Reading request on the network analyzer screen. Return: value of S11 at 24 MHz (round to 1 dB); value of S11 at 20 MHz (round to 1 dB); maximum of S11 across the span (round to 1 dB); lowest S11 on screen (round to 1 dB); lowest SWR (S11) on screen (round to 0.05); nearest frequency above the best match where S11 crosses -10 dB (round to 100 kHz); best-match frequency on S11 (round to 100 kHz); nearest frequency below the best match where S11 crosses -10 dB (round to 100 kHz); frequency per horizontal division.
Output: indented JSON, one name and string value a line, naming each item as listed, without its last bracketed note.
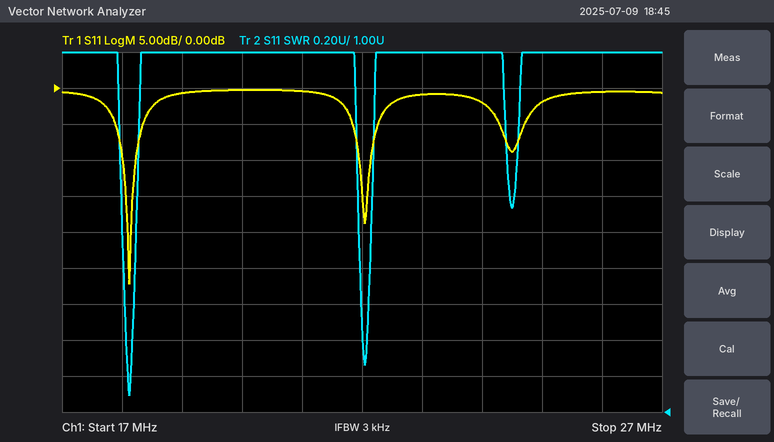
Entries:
{
  "value of S11 at 24 MHz": "-2 dB",
  "value of S11 at 20 MHz": "0 dB",
  "maximum of S11 across the span": "0 dB",
  "lowest S11 on screen": "-27 dB",
  "lowest SWR (S11) on screen": "1.10",
  "nearest frequency above the best match where S11 crosses -10 dB": "18.2 MHz",
  "best-match frequency on S11": "18.1 MHz",
  "nearest frequency below the best match where S11 crosses -10 dB": "18.0 MHz",
  "frequency per horizontal division": "1 MHz"
}
